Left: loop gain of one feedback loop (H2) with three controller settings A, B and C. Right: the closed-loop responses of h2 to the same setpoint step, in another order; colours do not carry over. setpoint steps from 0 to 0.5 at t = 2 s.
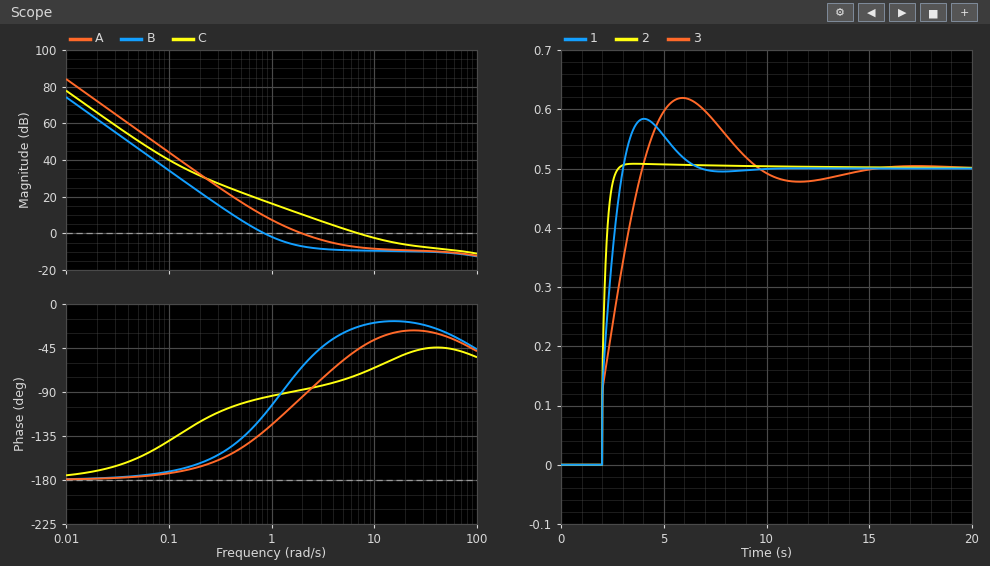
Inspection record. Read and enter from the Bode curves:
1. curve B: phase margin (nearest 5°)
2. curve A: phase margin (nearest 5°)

65°
85°
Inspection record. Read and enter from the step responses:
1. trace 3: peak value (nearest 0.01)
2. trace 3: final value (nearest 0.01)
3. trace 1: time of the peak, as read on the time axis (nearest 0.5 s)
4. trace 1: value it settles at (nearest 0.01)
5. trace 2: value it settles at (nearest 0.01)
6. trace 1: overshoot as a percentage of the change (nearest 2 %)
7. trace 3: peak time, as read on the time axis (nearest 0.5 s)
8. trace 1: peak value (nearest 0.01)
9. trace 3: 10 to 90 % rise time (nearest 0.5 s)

0.62
0.50
4.0 s
0.50
0.50
16 %
6.0 s
0.58
1.5 s
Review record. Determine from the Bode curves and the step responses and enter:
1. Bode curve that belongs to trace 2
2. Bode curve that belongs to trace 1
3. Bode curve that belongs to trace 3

C
A
B
